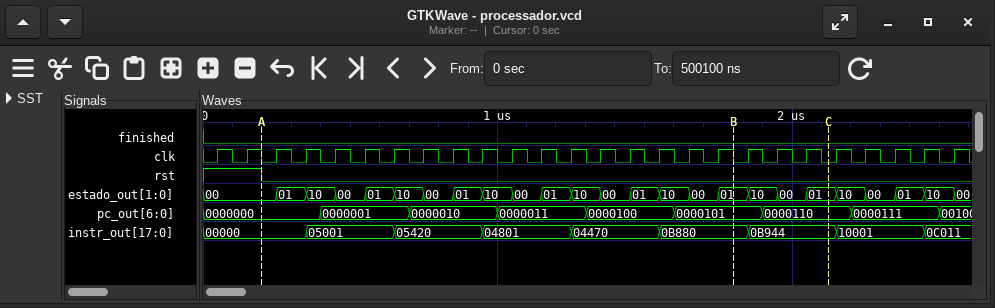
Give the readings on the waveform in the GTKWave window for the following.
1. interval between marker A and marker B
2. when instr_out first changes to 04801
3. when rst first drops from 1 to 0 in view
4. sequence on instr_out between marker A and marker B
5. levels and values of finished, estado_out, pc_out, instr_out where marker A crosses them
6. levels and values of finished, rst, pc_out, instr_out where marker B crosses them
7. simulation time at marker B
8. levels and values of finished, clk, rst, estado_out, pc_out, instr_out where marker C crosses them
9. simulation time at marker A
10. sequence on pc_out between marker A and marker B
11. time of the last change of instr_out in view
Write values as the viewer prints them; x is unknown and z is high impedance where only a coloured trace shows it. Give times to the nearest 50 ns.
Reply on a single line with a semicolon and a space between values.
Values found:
1600 ns; 950 ns; 200 ns; 00000, 05001, 05420, 04801, 04470, 0B880; finished=0, estado_out=00, pc_out=0000000, instr_out=00000; finished=0, rst=0, pc_out=0000101, instr_out=0B880; 1800 ns; finished=0, clk=0, rst=0, estado_out=01, pc_out=0000110, instr_out=0B944; 200 ns; 0000000, 0000001, 0000010, 0000011, 0000100, 0000101; 2450 ns
